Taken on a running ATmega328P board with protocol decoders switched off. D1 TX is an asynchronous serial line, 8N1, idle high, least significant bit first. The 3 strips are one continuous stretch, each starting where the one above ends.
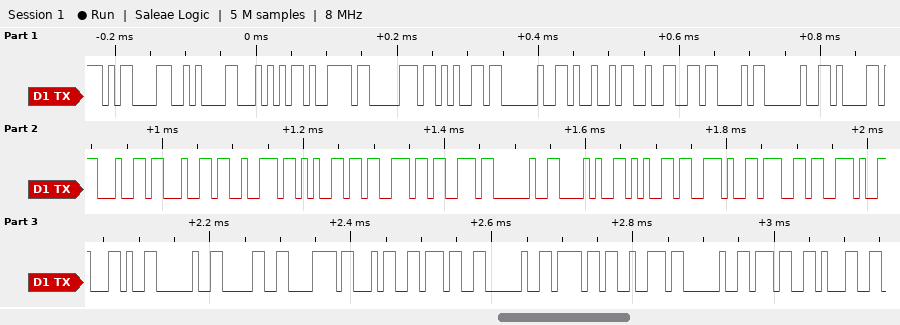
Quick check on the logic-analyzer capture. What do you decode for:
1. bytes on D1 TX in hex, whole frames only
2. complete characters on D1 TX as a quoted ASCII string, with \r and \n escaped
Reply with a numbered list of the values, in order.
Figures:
1. 0D 0A 54 79 70 65 20 49 32 43 20 61 64 64 72 65 73 73 20 28 65 2E 67 2E 2C 20 30 78 34 37 20 6F 72 20 37 31
2. "\r\nType I2C address (e.g., 0x47 or 71"
